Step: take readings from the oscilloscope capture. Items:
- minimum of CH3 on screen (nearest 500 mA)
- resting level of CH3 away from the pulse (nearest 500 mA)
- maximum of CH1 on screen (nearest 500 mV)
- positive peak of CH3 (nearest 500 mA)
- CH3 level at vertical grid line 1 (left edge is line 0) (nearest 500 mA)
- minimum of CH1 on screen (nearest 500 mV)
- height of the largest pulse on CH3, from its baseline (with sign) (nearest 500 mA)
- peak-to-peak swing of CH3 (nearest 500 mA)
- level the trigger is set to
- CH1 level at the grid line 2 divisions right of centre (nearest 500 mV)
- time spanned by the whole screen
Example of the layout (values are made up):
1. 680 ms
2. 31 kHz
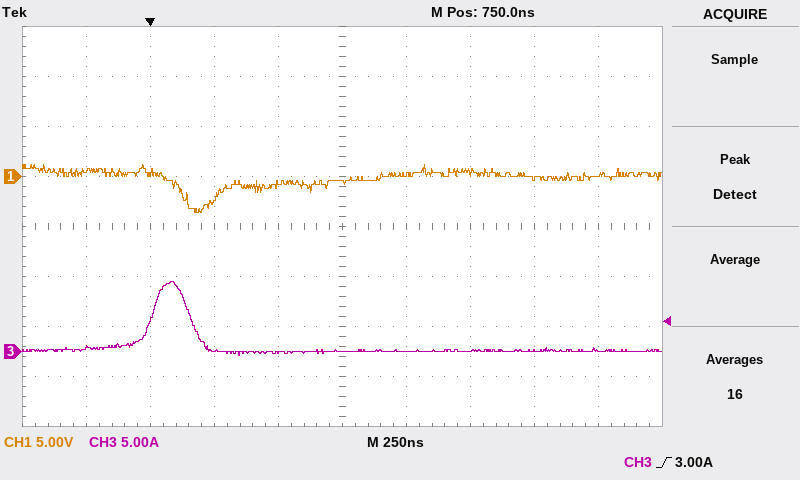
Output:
1. -500 mA
2. 0.0 A
3. 1.0 V
4. 7.0 A
5. 500 mA
6. -3.5 V
7. +7.0 A
8. 7.5 A
9. 3.00 A
10. 500 mV
11. 2.5 µs
